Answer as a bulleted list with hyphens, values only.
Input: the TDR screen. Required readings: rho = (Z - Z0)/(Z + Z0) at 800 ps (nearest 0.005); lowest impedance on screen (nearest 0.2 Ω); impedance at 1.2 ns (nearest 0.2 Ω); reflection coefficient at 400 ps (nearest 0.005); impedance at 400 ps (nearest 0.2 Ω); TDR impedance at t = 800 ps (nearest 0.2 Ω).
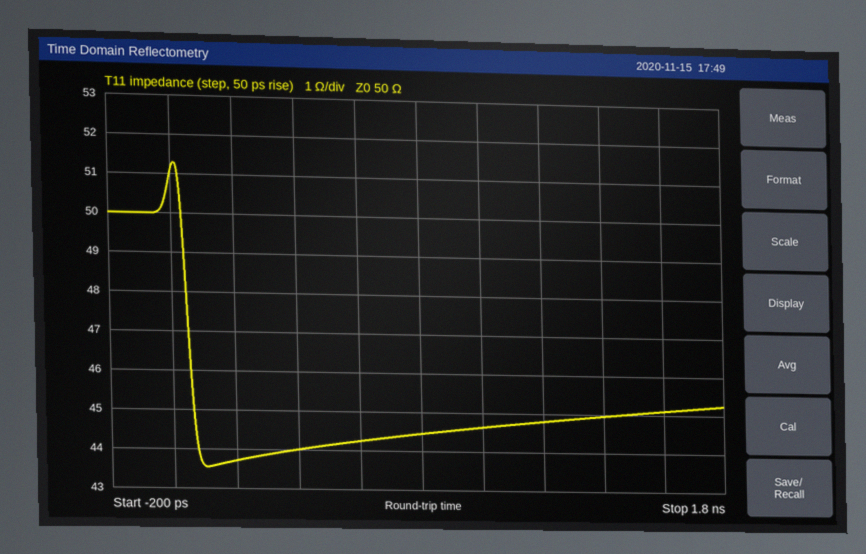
- -0.060
- 43.6 Ω
- 44.8 Ω
- -0.065
- 44.0 Ω
- 44.4 Ω
